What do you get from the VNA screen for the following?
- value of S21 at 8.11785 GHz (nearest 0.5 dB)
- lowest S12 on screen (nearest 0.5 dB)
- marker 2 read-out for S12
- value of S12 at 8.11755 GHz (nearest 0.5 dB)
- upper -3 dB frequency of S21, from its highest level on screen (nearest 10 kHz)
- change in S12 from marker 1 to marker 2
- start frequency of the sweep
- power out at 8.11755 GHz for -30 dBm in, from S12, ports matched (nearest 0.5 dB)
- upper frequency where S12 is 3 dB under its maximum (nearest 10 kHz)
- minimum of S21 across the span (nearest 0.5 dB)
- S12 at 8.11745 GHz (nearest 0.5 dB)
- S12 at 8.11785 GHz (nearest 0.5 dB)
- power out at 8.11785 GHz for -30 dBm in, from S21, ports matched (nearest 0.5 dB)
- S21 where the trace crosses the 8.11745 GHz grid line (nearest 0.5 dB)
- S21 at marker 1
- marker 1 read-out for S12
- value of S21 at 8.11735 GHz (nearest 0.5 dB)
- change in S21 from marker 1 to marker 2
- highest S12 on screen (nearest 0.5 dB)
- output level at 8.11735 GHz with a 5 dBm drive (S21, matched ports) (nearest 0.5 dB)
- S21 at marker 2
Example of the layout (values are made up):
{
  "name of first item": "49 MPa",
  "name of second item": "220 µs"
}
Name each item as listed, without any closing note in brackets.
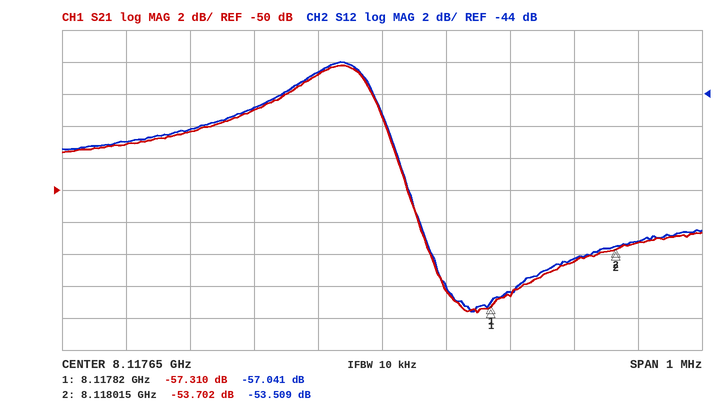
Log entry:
{
  "value of S21 at 8.11785 GHz": "-56.5 dB",
  "lowest S12 on screen": "-57.5 dB",
  "marker 2 read-out for S12": "-53.509 dB",
  "value of S12 at 8.11755 GHz": "-42.5 dB",
  "upper -3 dB frequency of S21, from its highest level on screen": "8.11765 GHz",
  "change in S12 from marker 1 to marker 2": "3.532 dB",
  "start frequency of the sweep": "8.11715 GHz",
  "power out at 8.11755 GHz for -30 dBm in, from S12, ports matched": "-72.5 dBm",
  "upper frequency where S12 is 3 dB under its maximum": "8.11765 GHz",
  "minimum of S21 across the span": "-57.5 dB",
  "S12 at 8.11745 GHz": "-45.0 dB",
  "S12 at 8.11785 GHz": "-56.5 dB",
  "power out at 8.11785 GHz for -30 dBm in, from S21, ports matched": "-86.5 dBm",
  "S21 where the trace crosses the 8.11745 GHz grid line": "-45.0 dB",
  "S21 at marker 1": "-57.310 dB",
  "marker 1 read-out for S12": "-57.041 dB",
  "value of S21 at 8.11735 GHz": "-46.5 dB",
  "change in S21 from marker 1 to marker 2": "3.608 dB",
  "highest S12 on screen": "-42.0 dB",
  "output level at 8.11735 GHz with a 5 dBm drive (S21, matched ports)": "-41.5 dBm",
  "S21 at marker 2": "-53.702 dB"
}
